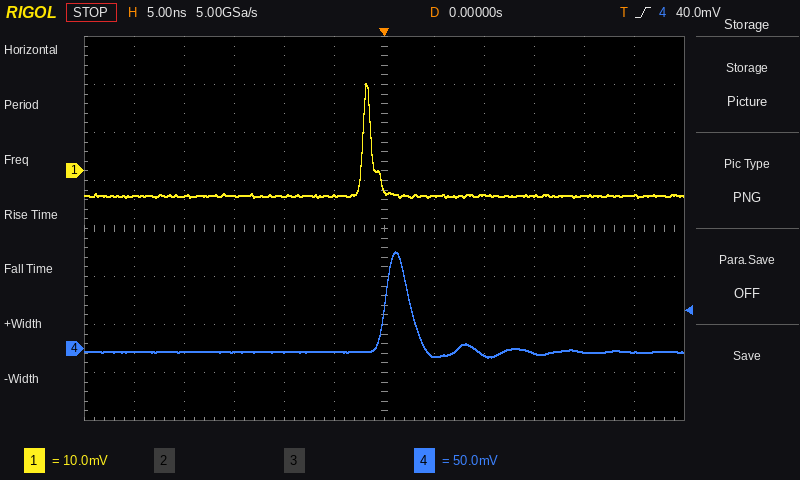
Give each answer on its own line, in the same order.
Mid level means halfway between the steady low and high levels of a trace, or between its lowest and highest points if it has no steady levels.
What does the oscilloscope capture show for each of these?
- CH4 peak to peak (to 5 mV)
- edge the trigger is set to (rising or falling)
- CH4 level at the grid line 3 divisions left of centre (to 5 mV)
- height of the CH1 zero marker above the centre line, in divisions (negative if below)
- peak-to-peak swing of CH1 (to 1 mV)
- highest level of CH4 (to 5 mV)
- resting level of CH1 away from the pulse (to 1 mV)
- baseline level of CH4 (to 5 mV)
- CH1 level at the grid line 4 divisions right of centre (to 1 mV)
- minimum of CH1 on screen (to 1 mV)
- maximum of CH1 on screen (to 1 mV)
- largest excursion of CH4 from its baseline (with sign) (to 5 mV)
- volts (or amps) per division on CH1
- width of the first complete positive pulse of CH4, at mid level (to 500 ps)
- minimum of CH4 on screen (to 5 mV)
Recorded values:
110 mV
rising
-5 mV
+1.2 div
24 mV
100 mV
-5 mV
-5 mV
-5 mV
-6 mV
18 mV
+105 mV
10 mV
2.5 ns
-10 mV
